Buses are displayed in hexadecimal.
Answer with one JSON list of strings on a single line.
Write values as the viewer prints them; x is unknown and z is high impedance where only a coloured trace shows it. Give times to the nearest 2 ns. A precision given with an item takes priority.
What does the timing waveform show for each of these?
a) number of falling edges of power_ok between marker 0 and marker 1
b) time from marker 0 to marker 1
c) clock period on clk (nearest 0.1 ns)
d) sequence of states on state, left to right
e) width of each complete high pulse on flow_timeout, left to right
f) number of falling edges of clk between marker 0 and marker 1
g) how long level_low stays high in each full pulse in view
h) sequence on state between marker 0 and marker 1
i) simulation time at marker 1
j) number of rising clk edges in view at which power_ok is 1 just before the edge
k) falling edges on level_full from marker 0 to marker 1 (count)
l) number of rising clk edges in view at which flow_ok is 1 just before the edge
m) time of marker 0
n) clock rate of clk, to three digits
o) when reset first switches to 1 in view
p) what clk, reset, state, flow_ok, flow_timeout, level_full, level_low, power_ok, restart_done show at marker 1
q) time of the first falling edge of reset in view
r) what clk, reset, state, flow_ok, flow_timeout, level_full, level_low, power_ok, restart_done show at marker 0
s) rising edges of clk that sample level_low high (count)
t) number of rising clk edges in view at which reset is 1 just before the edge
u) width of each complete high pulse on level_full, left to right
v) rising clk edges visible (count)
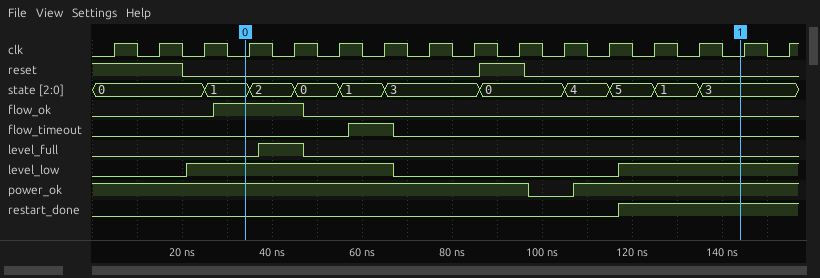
["1", "110 ns", "10 ns", "0, 1, 2, 0, 1, 3, 0, 4, 5, 1, 3", "10 ns", "11", "46 ns", "1, 2, 0, 1, 3, 0, 4, 5, 1, 3", "144 ns", "15", "1", "2", "34 ns", "100 MHz", "86 ns", "clk=0, reset=0, state=3, flow_ok=0, flow_timeout=0, level_full=0, level_low=1, power_ok=1, restart_done=1", "20 ns", "clk=0, reset=0, state=1, flow_ok=1, flow_timeout=0, level_full=0, level_low=1, power_ok=1, restart_done=0", "9", "3", "10 ns", "16"]
